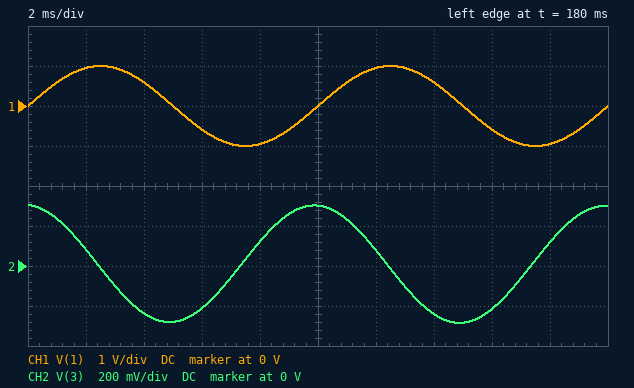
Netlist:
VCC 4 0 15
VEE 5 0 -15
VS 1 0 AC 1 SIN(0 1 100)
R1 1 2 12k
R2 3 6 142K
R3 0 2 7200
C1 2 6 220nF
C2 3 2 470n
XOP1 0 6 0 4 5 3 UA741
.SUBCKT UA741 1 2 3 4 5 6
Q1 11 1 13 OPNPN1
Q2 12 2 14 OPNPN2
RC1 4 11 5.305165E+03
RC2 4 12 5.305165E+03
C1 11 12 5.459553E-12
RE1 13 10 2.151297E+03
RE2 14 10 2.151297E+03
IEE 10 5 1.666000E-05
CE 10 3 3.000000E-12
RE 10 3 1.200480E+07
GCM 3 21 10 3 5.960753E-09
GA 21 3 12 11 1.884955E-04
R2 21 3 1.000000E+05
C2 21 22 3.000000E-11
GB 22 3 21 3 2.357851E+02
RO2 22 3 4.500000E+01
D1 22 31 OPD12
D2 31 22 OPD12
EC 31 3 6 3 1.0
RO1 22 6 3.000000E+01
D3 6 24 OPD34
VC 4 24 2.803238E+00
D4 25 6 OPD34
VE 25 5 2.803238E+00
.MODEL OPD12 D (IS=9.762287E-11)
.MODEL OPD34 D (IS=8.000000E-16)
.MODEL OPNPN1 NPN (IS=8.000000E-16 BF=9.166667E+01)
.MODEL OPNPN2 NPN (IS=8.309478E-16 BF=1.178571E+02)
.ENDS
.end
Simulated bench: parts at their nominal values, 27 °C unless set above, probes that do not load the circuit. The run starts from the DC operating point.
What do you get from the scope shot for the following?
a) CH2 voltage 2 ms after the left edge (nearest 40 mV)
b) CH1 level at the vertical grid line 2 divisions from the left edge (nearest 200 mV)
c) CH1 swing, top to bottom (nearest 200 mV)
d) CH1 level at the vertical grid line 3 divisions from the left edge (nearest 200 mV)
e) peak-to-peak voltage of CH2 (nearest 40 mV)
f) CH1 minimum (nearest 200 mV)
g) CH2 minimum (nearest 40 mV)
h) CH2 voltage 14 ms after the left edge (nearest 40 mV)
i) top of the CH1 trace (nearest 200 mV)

80 mV
600 mV
2.0 V
-600 mV
600 mV
-1.0 V
-280 mV
-240 mV
1.0 V
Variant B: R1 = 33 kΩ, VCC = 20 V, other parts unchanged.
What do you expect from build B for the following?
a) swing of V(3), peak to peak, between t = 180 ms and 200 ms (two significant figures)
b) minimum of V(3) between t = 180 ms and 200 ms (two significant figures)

210 mV
-98 mV
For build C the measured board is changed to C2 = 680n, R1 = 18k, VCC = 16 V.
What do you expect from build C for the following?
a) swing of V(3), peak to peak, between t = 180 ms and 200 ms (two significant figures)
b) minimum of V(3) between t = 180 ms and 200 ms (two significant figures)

270 mV
-130 mV
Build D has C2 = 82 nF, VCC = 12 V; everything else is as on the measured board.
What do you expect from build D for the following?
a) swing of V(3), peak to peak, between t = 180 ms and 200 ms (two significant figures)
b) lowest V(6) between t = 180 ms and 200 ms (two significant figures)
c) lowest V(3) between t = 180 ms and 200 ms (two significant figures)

4.0 V
-1.2 mV
-2.0 V
